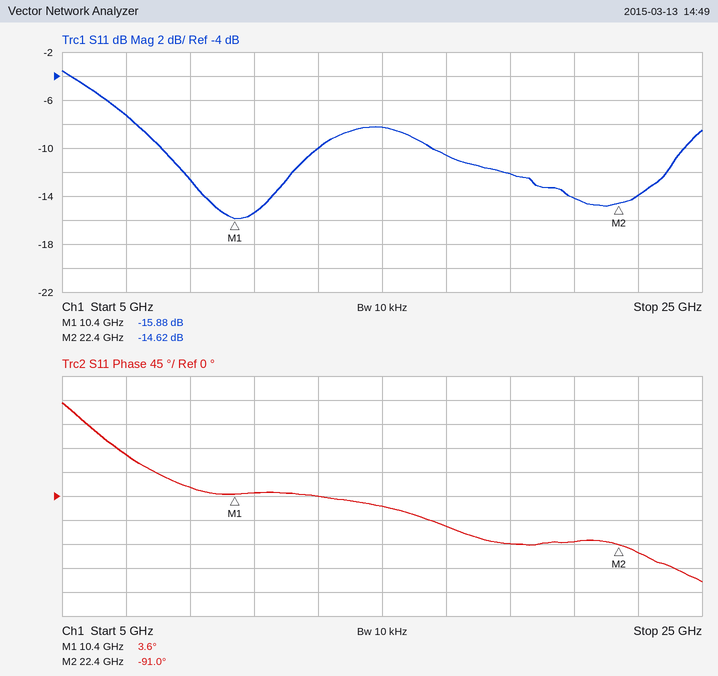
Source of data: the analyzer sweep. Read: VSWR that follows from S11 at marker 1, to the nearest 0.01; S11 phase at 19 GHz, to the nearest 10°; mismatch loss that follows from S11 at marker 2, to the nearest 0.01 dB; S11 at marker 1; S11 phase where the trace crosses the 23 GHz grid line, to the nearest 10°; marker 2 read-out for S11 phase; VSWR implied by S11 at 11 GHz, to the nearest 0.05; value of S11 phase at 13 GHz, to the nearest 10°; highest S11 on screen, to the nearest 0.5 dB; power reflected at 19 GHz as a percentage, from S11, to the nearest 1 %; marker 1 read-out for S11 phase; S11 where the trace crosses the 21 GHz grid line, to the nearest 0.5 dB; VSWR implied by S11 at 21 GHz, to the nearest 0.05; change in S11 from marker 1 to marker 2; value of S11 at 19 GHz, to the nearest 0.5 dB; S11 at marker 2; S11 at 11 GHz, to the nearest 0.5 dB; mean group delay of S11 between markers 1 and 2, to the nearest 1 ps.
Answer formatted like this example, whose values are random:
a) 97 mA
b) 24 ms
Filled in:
a) 1.38
b) -90°
c) 0.15 dB
d) -15.88 dB
e) -110°
f) -91.0°
g) 1.40
h) 0°
i) -3.5 dB
j) 6 %
k) 3.6°
l) -14.0 dB
m) 1.50
n) 1.26 dB
o) -12.0 dB
p) -14.62 dB
q) -15.5 dB
r) 22 ps
